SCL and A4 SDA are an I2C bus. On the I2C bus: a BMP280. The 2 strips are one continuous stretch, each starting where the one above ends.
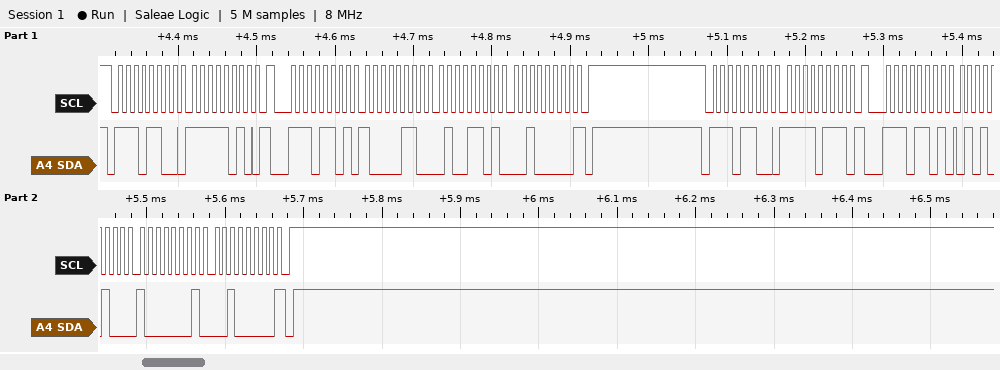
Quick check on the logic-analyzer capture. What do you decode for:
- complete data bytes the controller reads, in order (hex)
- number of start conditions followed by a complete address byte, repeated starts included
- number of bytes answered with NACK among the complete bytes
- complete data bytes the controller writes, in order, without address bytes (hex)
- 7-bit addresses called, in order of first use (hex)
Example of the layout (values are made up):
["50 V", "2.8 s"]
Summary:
["86 4D 20 54 81 20", "4", "2", "FA F7", "0x76"]
